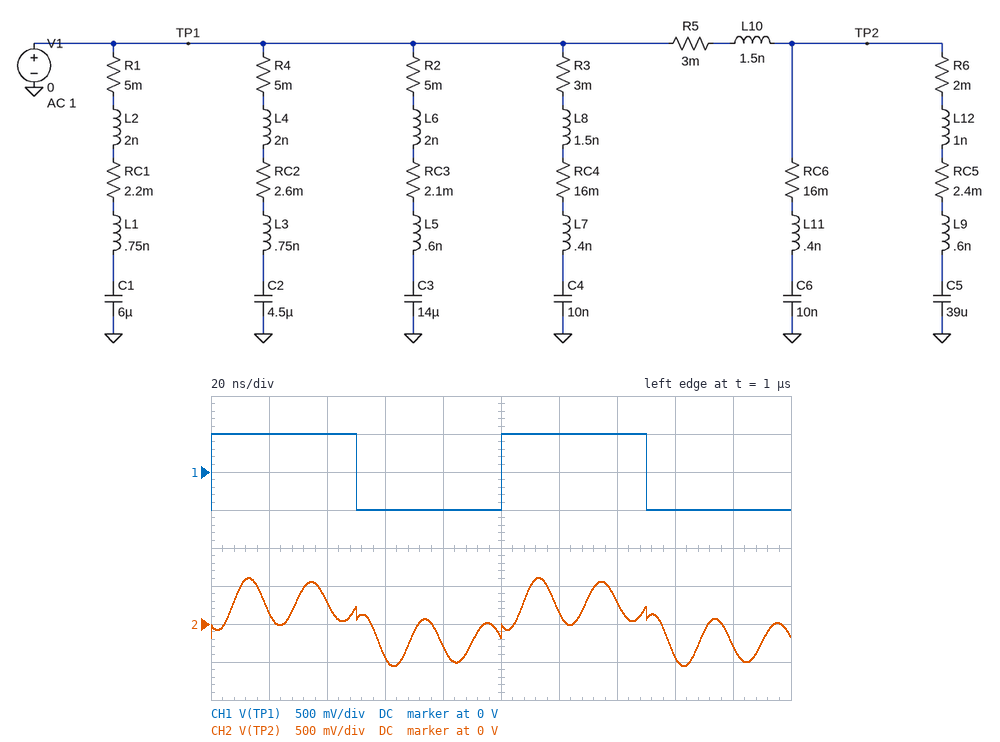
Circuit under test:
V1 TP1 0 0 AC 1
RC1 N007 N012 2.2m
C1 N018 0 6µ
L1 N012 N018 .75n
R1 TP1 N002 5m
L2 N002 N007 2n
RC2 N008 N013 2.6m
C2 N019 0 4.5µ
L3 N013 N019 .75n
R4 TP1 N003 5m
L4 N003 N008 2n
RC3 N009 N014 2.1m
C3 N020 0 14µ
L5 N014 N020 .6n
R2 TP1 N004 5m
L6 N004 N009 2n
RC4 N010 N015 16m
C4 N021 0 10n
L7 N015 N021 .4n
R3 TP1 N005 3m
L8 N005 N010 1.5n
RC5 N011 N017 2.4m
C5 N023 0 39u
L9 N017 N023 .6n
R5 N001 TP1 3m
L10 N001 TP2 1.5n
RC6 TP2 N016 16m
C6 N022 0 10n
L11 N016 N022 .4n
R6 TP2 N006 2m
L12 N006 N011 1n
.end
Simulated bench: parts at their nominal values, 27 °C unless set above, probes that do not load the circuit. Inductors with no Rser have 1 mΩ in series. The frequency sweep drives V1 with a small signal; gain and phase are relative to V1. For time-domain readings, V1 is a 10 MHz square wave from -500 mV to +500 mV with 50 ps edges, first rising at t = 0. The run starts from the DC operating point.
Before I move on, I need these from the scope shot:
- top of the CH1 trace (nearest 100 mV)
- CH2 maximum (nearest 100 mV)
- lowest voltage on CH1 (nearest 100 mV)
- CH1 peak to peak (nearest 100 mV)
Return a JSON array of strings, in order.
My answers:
["500 mV", "600 mV", "-500 mV", "1.0 V"]
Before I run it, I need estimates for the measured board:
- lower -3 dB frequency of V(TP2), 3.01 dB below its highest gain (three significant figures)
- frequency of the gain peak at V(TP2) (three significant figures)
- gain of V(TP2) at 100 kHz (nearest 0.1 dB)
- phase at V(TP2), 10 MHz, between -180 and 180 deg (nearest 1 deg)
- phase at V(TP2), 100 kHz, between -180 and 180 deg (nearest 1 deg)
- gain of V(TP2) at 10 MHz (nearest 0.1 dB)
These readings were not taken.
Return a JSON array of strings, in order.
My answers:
["45.0 MHz", "46.4 MHz", "0 dB", "-1 deg", "-6 deg", "-5.5 dB"]
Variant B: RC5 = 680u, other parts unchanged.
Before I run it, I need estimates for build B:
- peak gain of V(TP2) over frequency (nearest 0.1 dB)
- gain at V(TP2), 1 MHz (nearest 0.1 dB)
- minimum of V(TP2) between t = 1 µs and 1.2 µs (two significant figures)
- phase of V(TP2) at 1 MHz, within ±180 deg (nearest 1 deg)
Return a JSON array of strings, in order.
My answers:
["15.7 dB", "-7.3 dB", "-550 mV", "-9 deg"]
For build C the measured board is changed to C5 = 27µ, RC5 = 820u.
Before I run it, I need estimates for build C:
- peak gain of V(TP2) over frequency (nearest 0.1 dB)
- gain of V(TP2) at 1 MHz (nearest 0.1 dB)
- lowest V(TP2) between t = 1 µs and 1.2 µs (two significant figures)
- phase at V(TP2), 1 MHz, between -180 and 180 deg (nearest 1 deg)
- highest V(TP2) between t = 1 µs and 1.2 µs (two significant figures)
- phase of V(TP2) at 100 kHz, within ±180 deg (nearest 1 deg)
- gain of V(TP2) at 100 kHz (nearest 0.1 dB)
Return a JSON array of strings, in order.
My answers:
["15.7 dB", "-8.1 dB", "-540 mV", "-16 deg", "640 mV", "-4 deg", "0.1 dB"]
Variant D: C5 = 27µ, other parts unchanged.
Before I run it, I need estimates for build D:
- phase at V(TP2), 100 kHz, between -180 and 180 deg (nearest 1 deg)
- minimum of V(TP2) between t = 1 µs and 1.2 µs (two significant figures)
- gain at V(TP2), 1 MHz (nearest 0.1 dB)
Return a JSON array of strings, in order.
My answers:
["-4 deg", "-550 mV", "-7.0 dB"]
